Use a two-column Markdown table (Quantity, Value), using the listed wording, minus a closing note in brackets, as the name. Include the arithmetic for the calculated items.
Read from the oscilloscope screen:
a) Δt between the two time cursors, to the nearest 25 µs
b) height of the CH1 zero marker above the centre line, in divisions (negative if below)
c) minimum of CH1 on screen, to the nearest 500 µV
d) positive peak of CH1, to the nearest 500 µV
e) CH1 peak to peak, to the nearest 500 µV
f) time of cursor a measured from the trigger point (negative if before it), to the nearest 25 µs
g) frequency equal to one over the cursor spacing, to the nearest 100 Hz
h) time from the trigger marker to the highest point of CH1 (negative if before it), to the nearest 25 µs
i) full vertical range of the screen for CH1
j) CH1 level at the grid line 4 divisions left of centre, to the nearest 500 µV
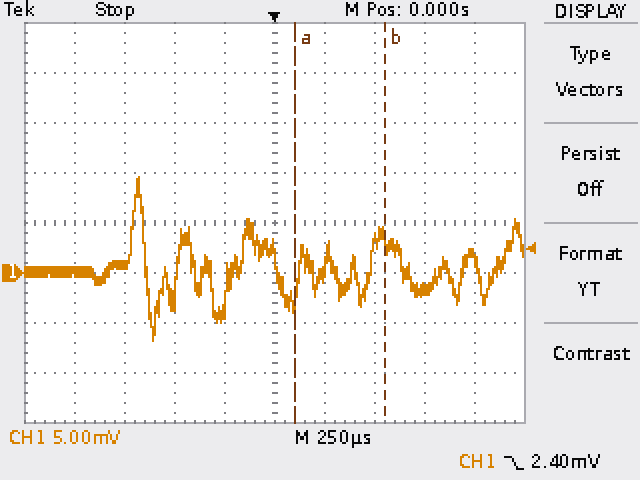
| Quantity | Value |
|---|---|
| Δt between the two time cursors, to the nearest 25 µs | 450 µs |
| height of the CH1 zero marker above the centre line, in divisions | -1.0 div |
| minimum of CH1 on screen, to the nearest 500 µV | -7.0 mV |
| positive peak of CH1, to the nearest 500 µV | 9.5 mV |
| CH1 peak to peak, to the nearest 500 µV | 9.5 mV − (-7.0 mV) = 16.5 mV |
| time of cursor a measured from the trigger point (negative if before it), to the nearest 25 µs | +100 µs |
| frequency equal to one over the cursor spacing, to the nearest 100 Hz | 1 / 450 µs ≈ 2.2 kHz |
| time from the trigger marker to the highest point of CH1 (negative if before it), to the nearest 25 µs | -675 µs |
| full vertical range of the screen for CH1 | 40 mV |
| CH1 level at the grid line 4 divisions left of centre, to the nearest 500 µV | 0.0 mV |
